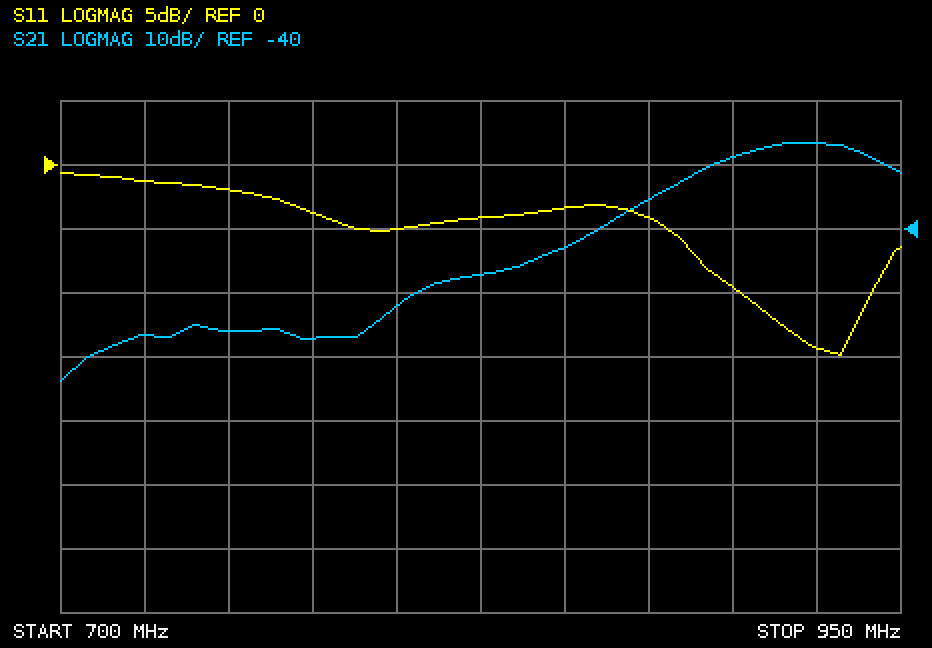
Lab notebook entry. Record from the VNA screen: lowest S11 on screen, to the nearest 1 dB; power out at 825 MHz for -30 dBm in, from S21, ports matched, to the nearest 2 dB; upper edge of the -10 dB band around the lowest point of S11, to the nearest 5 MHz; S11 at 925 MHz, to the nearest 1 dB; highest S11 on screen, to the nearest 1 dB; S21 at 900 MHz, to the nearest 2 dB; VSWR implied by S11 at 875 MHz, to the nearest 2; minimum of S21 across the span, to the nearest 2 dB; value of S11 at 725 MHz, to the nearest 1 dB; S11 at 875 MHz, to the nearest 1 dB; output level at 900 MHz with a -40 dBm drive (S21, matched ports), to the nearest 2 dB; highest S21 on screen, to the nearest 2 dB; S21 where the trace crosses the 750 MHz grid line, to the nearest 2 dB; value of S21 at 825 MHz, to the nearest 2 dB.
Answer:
-15 dB
-78 dBm
940 MHz
-14 dB
-1 dB
-28 dB
4
-64 dB
-1 dB
-4 dB
-68 dBm
-26 dB
-56 dB
-48 dB
